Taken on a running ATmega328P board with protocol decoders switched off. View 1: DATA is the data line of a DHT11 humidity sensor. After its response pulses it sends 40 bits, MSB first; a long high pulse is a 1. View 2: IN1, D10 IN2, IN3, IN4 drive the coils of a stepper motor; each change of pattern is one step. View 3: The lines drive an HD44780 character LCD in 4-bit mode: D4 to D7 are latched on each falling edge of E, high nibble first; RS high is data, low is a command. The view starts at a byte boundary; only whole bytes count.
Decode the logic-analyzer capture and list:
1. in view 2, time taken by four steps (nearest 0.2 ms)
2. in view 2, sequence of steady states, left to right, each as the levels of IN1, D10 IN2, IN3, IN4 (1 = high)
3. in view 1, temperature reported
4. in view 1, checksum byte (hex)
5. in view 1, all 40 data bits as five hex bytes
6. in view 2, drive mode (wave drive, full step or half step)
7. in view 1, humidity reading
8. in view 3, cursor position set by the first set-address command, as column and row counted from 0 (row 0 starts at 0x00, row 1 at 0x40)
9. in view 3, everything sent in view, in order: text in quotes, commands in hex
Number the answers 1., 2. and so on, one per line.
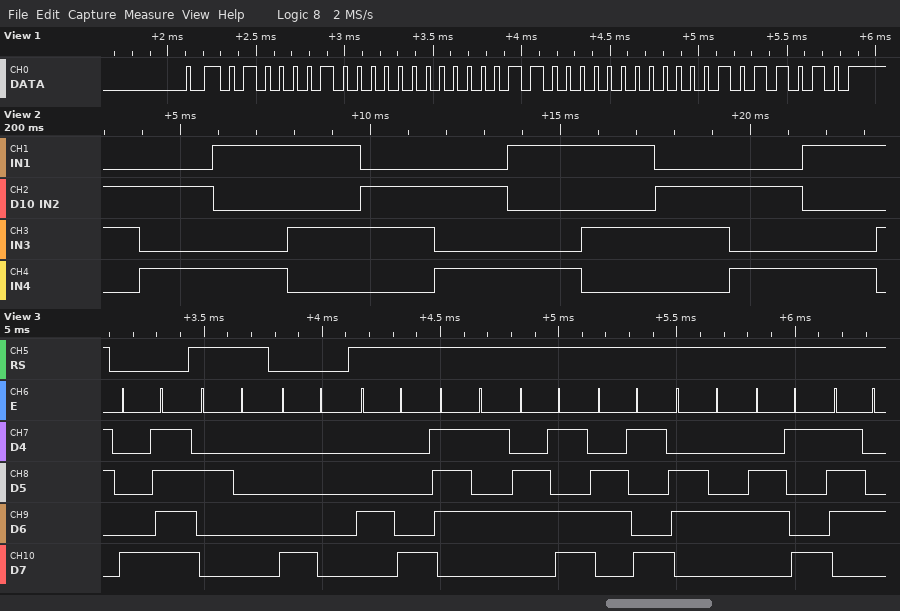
1. 7.8 ms
2. 0110 0101 1001 1010 0110 0101 1001 1010 0110 0101 1001 1010
3. 24.0 °C
4. 0x5A
5. 42 00 18 00 5A
6. full step
7. 66 %
8. column 15, row 0
9. 0x8F " " 0x80 "Humidit"
